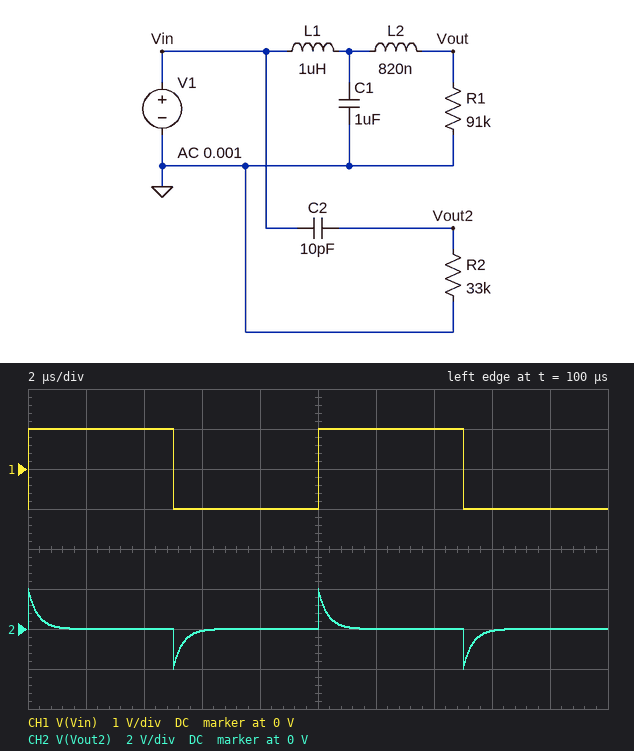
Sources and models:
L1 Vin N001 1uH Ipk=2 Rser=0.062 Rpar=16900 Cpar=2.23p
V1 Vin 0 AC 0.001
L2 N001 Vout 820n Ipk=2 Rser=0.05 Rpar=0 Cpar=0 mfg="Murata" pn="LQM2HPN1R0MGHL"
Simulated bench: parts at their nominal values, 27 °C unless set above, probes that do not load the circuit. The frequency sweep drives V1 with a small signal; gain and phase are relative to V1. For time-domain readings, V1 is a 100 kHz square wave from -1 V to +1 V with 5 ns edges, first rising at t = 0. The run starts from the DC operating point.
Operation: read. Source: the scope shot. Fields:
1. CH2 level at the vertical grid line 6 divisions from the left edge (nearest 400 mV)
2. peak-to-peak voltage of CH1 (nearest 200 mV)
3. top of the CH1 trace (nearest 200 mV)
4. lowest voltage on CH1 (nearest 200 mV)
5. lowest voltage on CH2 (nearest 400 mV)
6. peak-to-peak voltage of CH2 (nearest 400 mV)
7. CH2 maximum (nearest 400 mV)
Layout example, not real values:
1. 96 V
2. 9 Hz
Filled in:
1. 0 V
2. 2.0 V
3. 1.0 V
4. -1.0 V
5. -2.0 V
6. 4.0 V
7. 2.0 V
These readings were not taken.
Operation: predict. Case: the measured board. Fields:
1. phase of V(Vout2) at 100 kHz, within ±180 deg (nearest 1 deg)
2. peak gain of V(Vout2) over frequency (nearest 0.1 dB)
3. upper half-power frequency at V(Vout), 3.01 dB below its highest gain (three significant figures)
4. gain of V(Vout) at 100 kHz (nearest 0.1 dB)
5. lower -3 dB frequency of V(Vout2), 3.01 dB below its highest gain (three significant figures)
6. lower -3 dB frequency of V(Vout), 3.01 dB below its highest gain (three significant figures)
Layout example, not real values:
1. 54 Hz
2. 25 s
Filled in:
1. 78 deg
2. 0 dB
3. 164 kHz
4. 4.3 dB
5. 482 kHz
6. 154 kHz
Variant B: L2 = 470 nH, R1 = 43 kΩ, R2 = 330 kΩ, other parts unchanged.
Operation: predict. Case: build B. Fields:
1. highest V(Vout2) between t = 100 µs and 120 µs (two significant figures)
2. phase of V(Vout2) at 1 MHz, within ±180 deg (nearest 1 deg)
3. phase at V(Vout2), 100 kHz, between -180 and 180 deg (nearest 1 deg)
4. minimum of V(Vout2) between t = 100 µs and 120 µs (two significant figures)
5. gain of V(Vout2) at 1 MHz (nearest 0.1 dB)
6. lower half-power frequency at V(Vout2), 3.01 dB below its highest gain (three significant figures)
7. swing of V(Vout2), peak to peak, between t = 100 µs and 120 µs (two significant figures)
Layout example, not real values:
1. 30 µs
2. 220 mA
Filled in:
1. 1.6 V
2. 3 deg
3. 26 deg
4. -1.6 V
5. 0 dB
6. 48.2 kHz
7. 3.3 V
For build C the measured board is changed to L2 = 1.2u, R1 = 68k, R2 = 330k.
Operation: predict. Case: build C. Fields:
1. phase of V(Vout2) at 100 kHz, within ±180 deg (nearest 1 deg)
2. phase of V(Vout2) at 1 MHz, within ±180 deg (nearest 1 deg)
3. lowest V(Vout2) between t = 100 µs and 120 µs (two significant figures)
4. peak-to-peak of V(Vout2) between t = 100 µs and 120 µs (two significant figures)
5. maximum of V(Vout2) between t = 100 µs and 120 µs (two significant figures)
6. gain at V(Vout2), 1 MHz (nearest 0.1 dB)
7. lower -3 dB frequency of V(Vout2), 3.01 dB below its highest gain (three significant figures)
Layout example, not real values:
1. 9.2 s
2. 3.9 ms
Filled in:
1. 26 deg
2. 3 deg
3. -1.6 V
4. 3.3 V
5. 1.6 V
6. 0 dB
7. 48.2 kHz
